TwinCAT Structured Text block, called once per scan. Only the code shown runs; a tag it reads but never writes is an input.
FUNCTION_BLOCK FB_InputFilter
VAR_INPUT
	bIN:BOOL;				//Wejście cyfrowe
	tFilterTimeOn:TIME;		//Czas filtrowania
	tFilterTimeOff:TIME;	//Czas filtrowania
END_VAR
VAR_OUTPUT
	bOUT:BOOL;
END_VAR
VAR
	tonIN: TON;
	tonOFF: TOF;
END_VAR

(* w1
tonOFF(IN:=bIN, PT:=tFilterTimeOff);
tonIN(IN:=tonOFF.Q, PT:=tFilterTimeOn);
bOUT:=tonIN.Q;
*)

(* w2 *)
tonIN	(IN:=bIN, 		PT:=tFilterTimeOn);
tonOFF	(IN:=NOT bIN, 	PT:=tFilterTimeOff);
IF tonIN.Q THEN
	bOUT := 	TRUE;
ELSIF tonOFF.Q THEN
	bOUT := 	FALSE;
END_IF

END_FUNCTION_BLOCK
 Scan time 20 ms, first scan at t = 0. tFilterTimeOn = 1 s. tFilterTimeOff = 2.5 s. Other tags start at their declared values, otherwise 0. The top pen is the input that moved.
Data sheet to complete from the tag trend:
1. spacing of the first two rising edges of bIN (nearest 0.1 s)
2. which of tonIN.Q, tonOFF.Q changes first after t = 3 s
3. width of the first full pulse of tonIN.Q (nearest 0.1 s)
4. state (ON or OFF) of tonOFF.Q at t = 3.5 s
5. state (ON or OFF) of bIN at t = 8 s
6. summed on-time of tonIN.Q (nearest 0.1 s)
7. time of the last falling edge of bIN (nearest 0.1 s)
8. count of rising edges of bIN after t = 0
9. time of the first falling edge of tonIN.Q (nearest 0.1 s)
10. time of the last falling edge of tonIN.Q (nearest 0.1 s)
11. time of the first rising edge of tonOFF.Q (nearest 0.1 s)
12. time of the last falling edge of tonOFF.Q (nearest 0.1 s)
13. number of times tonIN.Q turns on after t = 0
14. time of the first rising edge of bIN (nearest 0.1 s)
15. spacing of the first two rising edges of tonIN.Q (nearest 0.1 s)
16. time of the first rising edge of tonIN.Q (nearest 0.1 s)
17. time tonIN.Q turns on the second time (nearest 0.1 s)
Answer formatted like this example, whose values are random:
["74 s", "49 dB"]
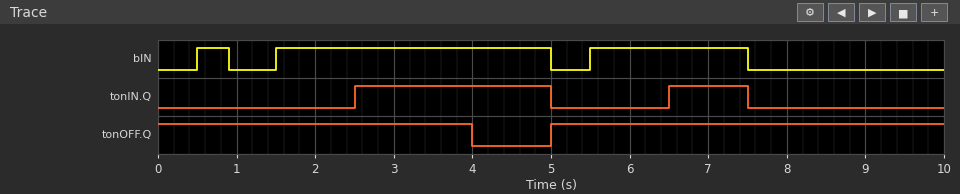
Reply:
["1.0 s", "tonOFF.Q", "2.5 s", "ON", "OFF", "3.5 s", "7.5 s", "3", "5.0 s", "7.5 s", "5.0 s", "4.0 s", "2", "0.5 s", "4.0 s", "2.5 s", "6.5 s"]
